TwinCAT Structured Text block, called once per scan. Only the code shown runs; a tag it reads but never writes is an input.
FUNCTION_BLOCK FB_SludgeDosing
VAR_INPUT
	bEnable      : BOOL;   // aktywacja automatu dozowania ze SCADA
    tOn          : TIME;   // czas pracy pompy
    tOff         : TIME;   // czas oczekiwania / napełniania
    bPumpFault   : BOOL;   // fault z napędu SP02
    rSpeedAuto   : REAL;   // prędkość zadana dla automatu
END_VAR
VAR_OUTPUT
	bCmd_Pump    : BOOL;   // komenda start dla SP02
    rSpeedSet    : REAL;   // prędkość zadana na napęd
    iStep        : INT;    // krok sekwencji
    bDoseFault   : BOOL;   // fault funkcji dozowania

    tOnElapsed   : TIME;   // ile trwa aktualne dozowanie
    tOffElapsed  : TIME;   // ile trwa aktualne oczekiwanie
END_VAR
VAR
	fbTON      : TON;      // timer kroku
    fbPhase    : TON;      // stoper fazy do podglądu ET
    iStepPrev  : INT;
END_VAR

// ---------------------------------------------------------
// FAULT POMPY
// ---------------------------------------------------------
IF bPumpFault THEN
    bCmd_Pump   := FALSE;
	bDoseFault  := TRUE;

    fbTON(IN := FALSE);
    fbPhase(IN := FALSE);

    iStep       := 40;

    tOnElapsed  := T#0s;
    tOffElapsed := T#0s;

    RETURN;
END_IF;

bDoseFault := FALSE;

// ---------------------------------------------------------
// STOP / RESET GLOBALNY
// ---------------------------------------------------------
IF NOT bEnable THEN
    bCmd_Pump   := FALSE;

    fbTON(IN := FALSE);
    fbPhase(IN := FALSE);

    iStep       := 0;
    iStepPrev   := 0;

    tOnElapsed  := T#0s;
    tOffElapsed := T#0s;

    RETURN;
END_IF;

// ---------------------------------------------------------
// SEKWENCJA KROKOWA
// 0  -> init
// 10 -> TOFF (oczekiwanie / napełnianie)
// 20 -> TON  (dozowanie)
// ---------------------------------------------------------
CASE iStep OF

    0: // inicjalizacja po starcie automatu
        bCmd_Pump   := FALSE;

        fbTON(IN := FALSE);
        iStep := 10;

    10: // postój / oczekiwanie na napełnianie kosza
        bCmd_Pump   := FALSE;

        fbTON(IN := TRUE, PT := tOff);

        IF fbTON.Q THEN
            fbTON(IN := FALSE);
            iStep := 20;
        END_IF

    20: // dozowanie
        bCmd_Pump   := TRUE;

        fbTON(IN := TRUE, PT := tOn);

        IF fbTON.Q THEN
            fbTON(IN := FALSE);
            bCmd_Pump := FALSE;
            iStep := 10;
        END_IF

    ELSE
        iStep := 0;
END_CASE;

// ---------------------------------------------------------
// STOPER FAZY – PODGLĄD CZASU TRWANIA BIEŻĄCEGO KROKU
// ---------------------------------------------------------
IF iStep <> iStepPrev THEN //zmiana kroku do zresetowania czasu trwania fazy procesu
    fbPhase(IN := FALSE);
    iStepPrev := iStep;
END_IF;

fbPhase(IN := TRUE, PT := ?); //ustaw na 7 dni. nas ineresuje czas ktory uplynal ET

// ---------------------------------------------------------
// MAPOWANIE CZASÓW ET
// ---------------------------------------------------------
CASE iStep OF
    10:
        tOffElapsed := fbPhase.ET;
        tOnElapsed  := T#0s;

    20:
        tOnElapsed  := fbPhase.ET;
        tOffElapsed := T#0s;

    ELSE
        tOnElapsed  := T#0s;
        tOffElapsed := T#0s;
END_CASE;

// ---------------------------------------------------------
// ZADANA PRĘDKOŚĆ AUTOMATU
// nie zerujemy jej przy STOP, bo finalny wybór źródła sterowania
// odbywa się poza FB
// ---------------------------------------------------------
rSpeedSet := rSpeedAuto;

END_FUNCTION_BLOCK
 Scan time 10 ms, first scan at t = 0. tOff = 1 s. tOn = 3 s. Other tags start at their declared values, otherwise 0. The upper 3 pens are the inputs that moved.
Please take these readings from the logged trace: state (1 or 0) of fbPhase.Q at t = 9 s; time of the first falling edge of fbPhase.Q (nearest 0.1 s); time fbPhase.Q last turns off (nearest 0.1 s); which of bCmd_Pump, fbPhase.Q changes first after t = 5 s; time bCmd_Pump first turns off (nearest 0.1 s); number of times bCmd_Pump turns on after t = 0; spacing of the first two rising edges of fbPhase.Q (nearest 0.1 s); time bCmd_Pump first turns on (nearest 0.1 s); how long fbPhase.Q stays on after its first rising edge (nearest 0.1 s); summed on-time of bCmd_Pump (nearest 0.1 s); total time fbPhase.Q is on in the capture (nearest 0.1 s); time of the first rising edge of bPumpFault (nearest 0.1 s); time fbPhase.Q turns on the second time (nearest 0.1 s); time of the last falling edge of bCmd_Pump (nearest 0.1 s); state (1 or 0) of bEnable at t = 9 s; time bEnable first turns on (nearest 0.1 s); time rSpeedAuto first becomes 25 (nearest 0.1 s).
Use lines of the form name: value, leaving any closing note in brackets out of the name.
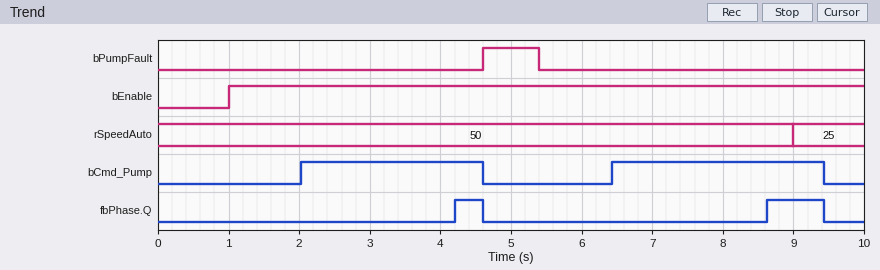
state (1 or 0) of fbPhase.Q at t = 9 s: 1
time of the first falling edge of fbPhase.Q: 4.6 s
time fbPhase.Q last turns off: 9.4 s
which of bCmd_Pump, fbPhase.Q changes first after t = 5 s: bCmd_Pump
time bCmd_Pump first turns off: 4.6 s
number of times bCmd_Pump turns on after t = 0: 2
spacing of the first two rising edges of fbPhase.Q: 4.4 s
time bCmd_Pump first turns on: 2.0 s
how long fbPhase.Q stays on after its first rising edge: 0.4 s
summed on-time of bCmd_Pump: 5.6 s
total time fbPhase.Q is on in the capture: 1.2 s
time of the first rising edge of bPumpFault: 4.6 s
time fbPhase.Q turns on the second time: 8.6 s
time of the last falling edge of bCmd_Pump: 9.4 s
state (1 or 0) of bEnable at t = 9 s: 1
time bEnable first turns on: 1.0 s
time rSpeedAuto first becomes 25: 9.0 s
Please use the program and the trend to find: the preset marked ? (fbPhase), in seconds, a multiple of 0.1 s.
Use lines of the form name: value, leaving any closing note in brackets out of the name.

the preset marked ? (fbPhase), in seconds, a multiple of 0.1 s: 2.2 s
